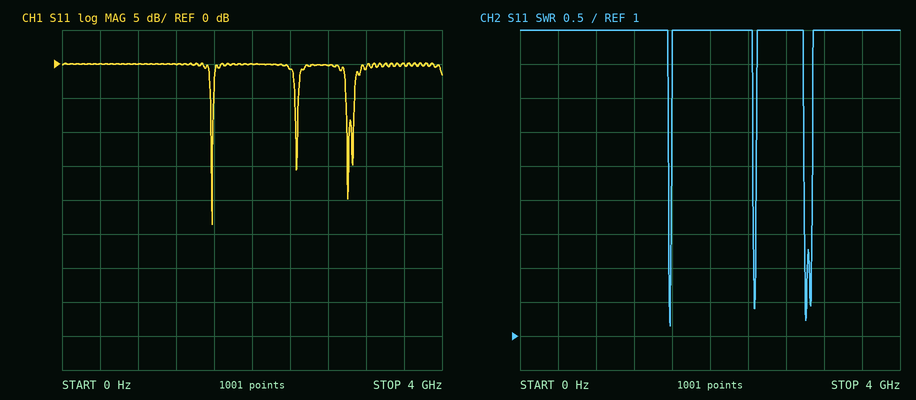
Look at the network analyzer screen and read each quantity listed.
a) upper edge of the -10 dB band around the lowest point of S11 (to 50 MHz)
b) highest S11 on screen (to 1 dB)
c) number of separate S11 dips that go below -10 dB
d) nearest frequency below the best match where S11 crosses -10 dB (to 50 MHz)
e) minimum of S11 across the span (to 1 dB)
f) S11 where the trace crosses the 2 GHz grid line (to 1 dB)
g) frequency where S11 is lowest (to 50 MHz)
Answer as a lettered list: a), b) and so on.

a) 1.60 GHz
b) 0 dB
c) 4
d) 1.55 GHz
e) -24 dB
f) 0 dB
g) 1.60 GHz
